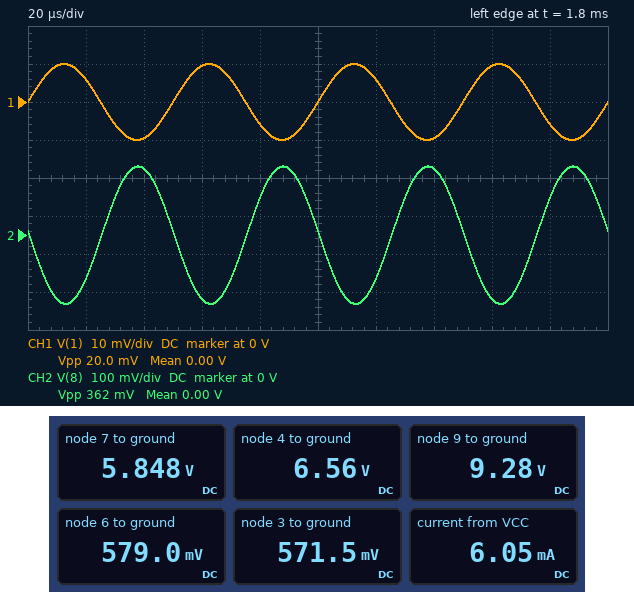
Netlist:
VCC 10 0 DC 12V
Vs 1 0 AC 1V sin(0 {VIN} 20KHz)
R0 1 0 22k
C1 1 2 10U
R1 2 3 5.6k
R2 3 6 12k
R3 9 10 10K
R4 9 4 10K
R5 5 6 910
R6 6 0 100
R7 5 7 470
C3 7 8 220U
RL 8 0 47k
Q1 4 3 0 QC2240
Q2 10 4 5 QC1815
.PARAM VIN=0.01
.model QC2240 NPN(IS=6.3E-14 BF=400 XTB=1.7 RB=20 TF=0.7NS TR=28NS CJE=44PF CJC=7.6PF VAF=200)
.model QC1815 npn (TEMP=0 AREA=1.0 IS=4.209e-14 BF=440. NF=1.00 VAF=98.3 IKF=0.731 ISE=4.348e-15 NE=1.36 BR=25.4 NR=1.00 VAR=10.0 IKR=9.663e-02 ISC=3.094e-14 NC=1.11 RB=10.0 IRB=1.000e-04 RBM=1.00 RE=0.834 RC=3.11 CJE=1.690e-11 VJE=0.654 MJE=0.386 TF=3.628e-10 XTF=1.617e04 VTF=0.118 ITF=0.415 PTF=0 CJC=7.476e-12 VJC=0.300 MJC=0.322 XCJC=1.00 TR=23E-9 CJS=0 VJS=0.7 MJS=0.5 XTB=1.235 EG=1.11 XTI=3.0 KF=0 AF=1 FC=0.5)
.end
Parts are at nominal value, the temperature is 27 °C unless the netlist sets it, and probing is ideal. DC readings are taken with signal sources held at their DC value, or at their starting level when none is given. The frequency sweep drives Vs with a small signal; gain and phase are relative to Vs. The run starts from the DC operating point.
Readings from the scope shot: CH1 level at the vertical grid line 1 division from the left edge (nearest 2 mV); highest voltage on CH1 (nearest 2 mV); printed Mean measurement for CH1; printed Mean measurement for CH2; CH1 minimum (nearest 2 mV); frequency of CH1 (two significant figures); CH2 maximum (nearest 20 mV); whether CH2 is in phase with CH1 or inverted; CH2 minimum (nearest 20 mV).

6 mV
10 mV
0.00 V
0.00 V
-10 mV
20 kHz
180 mV
inverted
-180 mV
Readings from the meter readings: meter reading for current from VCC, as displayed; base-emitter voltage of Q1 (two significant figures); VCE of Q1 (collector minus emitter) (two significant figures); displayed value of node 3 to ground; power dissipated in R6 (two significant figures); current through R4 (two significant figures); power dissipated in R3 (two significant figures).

6.05 mA
570 mV
6.6 V
571.5 mV
3.4 mW
270 µA
740 µW
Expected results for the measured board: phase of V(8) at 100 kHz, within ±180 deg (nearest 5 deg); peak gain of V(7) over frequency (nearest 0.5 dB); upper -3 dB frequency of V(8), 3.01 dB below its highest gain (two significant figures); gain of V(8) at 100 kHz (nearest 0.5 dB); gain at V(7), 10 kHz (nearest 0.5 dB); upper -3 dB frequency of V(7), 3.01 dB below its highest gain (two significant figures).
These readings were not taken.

165 deg
25.0 dB
370 kHz
25.0 dB
25.0 dB
370 kHz
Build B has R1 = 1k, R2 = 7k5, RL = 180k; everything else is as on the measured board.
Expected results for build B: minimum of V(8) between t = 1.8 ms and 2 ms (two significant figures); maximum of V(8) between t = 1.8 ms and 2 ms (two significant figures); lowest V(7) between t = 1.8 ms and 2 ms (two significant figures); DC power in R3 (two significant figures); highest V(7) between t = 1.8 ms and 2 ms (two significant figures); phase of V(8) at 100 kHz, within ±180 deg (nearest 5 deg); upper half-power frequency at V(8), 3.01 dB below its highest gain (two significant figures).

-520 mV
510 mV
5.3 V
750 µW
6.3 V
170 deg
640 kHz
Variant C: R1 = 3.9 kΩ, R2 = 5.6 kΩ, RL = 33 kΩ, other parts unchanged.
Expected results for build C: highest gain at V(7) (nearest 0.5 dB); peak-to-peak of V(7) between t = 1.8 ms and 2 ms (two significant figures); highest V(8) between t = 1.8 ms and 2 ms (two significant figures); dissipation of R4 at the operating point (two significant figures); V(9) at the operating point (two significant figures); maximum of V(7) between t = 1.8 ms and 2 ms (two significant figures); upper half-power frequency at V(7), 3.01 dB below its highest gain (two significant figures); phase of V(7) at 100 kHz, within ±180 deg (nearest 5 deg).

22.0 dB
250 mV
130 mV
750 µW
9.3 V
5.9 V
750 kHz
170 deg
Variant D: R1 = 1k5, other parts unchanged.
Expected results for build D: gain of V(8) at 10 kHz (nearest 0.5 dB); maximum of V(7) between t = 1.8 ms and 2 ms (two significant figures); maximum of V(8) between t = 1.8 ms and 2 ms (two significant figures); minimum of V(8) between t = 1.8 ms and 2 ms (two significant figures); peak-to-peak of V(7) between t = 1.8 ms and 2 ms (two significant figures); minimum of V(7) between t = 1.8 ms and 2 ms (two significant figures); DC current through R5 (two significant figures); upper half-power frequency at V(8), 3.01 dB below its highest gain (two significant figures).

34.5 dB
6.4 V
520 mV
-540 mV
1.1 V
5.3 V
5.8 mA
430 kHz
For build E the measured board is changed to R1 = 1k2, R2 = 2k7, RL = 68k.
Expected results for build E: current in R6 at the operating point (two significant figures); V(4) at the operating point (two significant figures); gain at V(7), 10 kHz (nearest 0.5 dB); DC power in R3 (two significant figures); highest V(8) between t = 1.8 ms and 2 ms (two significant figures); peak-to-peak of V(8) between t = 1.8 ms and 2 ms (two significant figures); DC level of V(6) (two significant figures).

5.7 mA
6.5 V
26.0 dB
750 µW
200 mV
390 mV
570 mV
